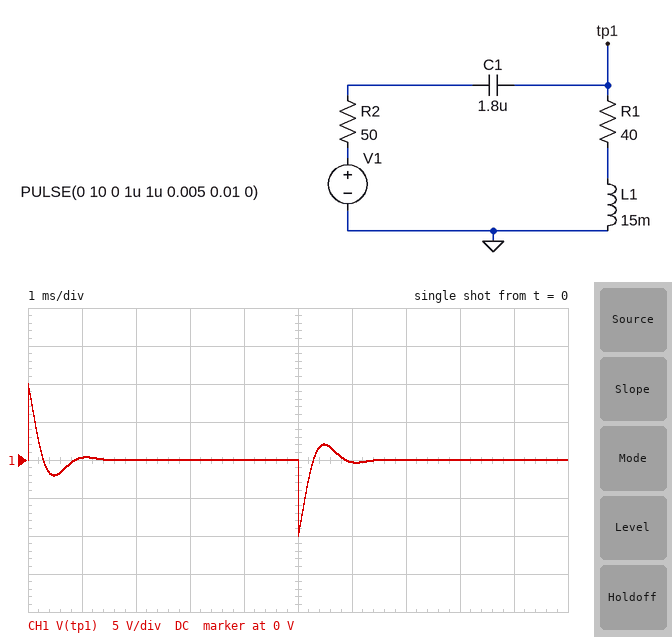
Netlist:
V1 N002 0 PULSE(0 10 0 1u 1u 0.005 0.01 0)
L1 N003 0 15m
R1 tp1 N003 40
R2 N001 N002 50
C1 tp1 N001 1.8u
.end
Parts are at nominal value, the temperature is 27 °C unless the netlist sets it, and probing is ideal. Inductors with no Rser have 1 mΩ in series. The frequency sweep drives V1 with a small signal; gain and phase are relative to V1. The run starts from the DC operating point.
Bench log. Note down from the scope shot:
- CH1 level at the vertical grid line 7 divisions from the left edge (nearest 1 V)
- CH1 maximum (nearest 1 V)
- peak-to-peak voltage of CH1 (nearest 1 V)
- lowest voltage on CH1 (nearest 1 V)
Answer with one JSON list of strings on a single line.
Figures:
["0 V", "10 V", "20 V", "-10 V"]
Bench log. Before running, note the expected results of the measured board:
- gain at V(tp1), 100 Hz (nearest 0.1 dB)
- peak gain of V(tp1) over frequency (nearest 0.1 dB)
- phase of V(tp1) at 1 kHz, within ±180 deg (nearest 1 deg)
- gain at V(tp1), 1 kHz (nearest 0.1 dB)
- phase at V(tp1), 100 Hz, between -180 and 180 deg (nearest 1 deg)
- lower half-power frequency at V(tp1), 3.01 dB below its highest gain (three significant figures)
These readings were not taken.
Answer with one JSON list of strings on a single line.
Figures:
["-26.6 dB", "1.8 dB", "63 deg", "1.1 dB", "97 deg", "790 Hz"]
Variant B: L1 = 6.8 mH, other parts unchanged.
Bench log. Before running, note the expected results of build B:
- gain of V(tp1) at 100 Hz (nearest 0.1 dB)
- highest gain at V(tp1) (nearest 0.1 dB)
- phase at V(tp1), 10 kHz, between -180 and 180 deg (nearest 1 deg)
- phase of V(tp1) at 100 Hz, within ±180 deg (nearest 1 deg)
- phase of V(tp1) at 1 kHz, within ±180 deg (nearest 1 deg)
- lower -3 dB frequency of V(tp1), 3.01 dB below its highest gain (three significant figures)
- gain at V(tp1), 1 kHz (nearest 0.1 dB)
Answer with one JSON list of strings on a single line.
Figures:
["-26.8 dB", "0.1 dB", "7 deg", "90 deg", "74 deg", "1.22 kHz", "-4.7 dB"]
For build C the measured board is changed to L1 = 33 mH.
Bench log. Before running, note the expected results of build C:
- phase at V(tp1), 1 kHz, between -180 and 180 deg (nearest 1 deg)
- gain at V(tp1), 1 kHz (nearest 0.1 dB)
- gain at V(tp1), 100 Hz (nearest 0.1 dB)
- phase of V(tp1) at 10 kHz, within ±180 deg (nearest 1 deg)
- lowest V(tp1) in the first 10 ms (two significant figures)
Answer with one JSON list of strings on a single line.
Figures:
["26 deg", "3.0 dB", "-25.7 dB", "1 deg", "-10 V"]
